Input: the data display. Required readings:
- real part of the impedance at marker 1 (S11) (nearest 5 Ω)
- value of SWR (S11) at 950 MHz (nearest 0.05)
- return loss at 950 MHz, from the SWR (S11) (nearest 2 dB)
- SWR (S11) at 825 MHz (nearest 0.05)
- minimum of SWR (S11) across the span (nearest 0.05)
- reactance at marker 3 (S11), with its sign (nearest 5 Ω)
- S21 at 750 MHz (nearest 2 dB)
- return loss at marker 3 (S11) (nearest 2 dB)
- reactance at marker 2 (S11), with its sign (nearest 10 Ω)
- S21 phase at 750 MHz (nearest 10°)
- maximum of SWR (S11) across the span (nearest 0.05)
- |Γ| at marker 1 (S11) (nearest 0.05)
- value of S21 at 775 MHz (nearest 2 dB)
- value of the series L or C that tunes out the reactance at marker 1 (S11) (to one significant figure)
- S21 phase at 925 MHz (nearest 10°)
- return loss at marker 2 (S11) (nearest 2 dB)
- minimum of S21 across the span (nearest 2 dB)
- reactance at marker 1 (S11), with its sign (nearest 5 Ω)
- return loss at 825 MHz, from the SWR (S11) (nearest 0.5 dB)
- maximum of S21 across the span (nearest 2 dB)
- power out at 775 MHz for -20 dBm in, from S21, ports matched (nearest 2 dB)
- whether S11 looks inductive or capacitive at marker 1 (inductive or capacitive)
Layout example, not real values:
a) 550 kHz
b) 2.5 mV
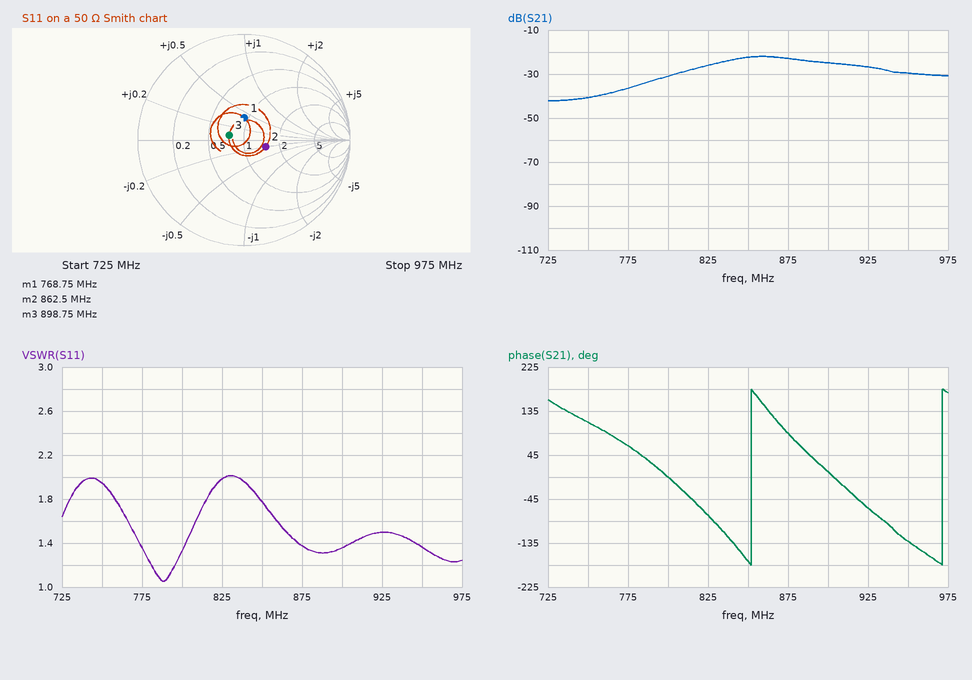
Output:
a) 45 Ω
b) 1.35
c) 16 dB
d) 2.00
e) 1.05
f) +5 Ω
g) -40 dB
h) 16 dB
i) -10 Ω
j) 110°
k) 2.00
l) 0.20
m) -36 dB
n) 10 pF
o) -60°
p) 14 dB
q) -42 dB
r) +20 Ω
s) 9.5 dB
t) -22 dB
u) -56 dBm
v) inductive
